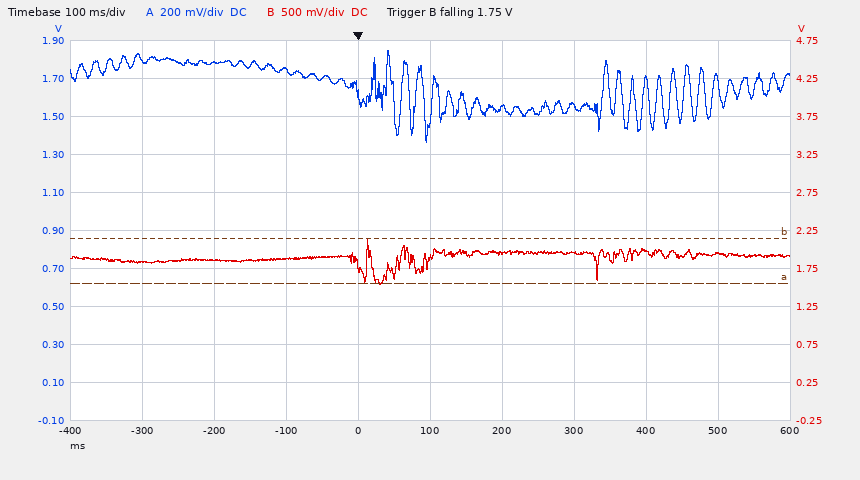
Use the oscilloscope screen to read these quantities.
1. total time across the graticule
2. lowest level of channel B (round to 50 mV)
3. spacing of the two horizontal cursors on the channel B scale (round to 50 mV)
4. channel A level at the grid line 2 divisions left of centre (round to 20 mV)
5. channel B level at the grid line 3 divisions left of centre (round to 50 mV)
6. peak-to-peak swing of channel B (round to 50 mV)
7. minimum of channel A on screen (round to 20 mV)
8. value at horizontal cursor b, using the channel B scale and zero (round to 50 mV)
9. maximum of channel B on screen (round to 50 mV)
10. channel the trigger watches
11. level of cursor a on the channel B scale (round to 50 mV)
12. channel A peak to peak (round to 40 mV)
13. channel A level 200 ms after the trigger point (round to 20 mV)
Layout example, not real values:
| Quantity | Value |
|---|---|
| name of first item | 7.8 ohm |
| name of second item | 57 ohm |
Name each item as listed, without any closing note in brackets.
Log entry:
| Quantity | Value |
|---|---|
| total time across the graticule | 1 s |
| lowest level of channel B | 1.55 V |
| spacing of the two horizontal cursors on the channel B scale | 600 mV |
| channel A level at the grid line 2 divisions left of centre | 1.74 V |
| channel B level at the grid line 3 divisions left of centre | 1.85 V |
| peak-to-peak swing of channel B | 600 mV |
| minimum of channel A on screen | 1.36 V |
| value at horizontal cursor b, using the channel B scale and zero | 2.15 V |
| maximum of channel B on screen | 2.15 V |
| channel the trigger watches | channel B |
| level of cursor a on the channel B scale | 1.55 V |
| channel A peak to peak | 480 mV |
| channel A level 200 ms after the trigger point | 1.54 V |
